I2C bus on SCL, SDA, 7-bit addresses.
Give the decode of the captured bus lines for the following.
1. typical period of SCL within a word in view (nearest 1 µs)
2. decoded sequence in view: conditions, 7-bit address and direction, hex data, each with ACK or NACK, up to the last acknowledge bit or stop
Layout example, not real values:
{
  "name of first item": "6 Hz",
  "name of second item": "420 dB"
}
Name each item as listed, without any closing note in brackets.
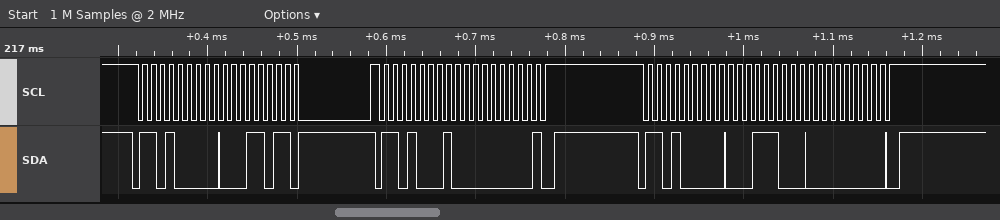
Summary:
{
  "typical period of SCL within a word in view": "10 µs",
  "decoded sequence in view: conditions, 7-bit address and direction, hex data, each with ACK or NACK, up to the last acknowledge bit or stop": "start, address 68 write ACK, 1B ACK, repeated start, address 68 read ACK, 00 NACK, stop, start, address 68 write ACK, 1C ACK, 00 ACK, stop"
}
